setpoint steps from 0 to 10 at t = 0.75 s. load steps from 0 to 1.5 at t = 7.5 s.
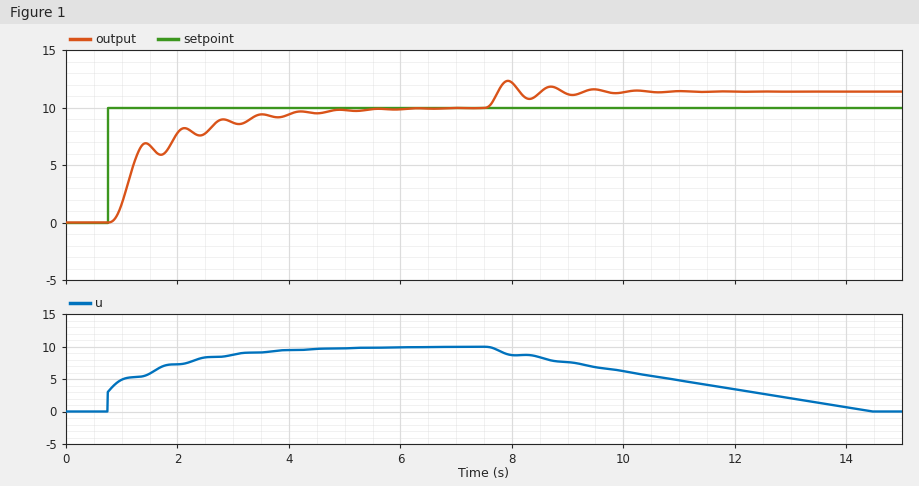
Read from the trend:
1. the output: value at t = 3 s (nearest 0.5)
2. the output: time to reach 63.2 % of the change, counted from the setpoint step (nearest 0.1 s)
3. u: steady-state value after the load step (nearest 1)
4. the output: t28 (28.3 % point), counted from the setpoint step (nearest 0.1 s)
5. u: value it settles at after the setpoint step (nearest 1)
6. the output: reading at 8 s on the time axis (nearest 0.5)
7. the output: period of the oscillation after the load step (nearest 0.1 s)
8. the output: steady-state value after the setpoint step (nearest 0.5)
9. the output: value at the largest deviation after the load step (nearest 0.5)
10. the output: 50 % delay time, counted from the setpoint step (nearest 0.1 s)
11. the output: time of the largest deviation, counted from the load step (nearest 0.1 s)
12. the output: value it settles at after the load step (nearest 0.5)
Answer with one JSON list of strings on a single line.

["8.5", "0.6 s", "0", "0.3 s", "10", "12.0", "0.8 s", "10.0", "12.5", "0.5 s", "0.4 s", "11.5"]
